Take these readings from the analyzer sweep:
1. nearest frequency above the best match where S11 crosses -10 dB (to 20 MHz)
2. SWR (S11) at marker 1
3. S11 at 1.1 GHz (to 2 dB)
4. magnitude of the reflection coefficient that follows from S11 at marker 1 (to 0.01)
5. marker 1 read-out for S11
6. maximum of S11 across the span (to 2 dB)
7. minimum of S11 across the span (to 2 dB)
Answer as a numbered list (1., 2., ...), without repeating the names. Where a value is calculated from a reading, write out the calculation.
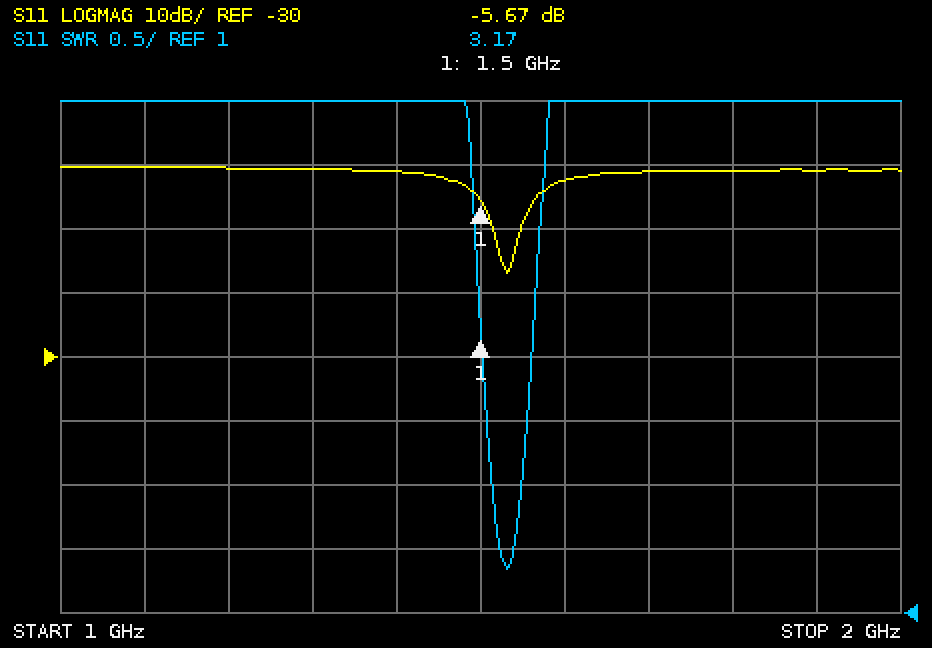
1. 1.54 GHz
2. 3.17
3. 0 dB
4. 10^(-5.67/20) ≈ 0.52
5. -5.67 dB
6. 0 dB
7. -16 dB
